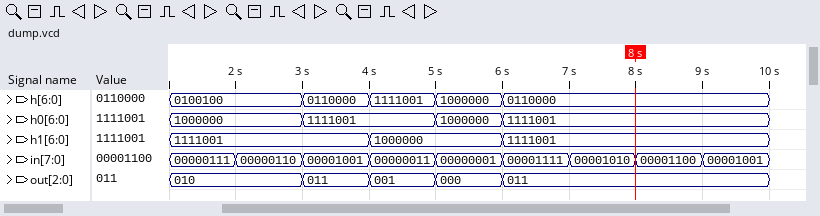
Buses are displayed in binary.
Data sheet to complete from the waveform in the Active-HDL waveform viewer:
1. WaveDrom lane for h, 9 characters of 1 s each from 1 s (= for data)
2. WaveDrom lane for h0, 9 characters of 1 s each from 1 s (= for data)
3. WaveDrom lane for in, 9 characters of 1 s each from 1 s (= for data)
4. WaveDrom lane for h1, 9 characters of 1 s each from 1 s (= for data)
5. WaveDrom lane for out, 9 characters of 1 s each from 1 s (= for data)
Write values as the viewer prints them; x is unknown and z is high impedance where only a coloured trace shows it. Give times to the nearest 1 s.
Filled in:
{name: 'h', wave: '=.====...', data: '0100100 0110000 1111001 1000000 0110000'}
{name: 'h0', wave: '=.=.==...', data: '1000000 1111001 1000000 1111001'}
{name: 'in', wave: '=========', data: '00000111 00000110 00001001 00000011 00000001 00001111 00001010 00001100 00001001'}
{name: 'h1', wave: '=..=.=...', data: '1111001 1000000 1111001'}
{name: 'out', wave: '=.====...', data: '010 011 001 000 011'}
